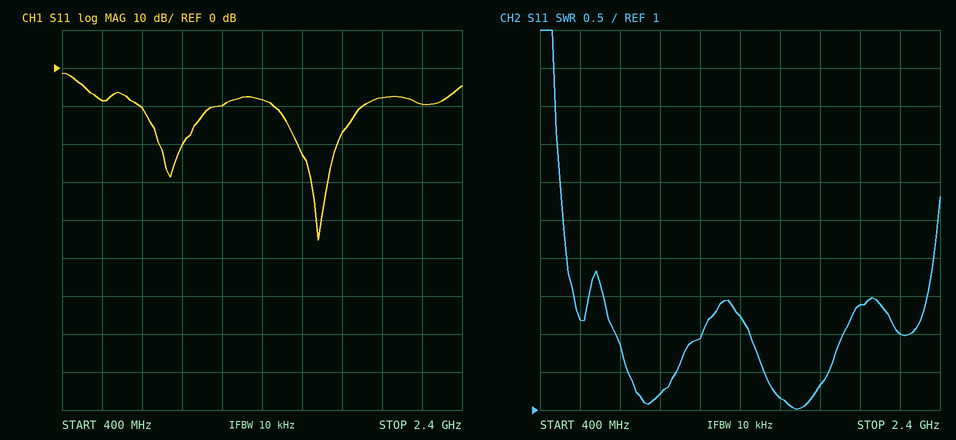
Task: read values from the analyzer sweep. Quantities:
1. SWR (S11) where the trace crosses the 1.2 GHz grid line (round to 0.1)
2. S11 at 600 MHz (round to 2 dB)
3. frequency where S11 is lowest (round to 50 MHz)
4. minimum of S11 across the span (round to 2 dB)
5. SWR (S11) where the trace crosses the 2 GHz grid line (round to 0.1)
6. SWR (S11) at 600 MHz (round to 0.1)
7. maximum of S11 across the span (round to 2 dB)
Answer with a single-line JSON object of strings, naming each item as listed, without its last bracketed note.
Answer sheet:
{"SWR (S11) where the trace crosses the 1.2 GHz grid line": "1.9", "S11 at 600 MHz": "-8 dB", "frequency where S11 is lowest": "1.70 GHz", "minimum of S11 across the span": "-46 dB", "SWR (S11) where the trace crosses the 2 GHz grid line": "2.4", "SWR (S11) at 600 MHz": "2.2", "maximum of S11 across the span": "-2 dB"}
